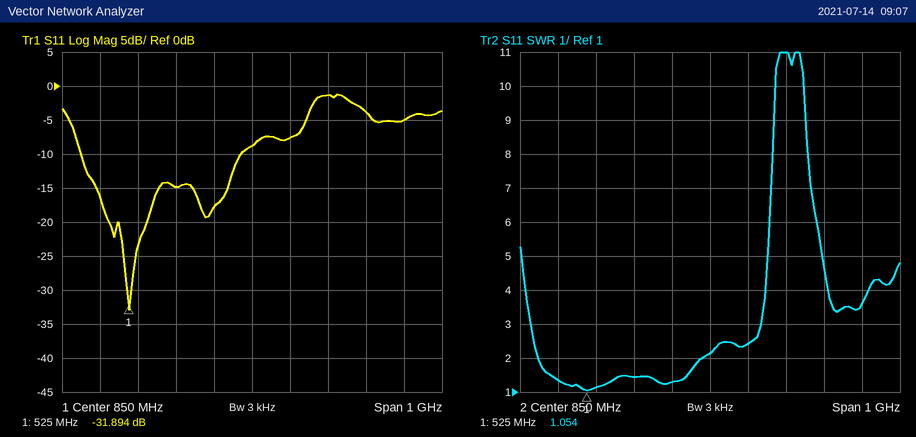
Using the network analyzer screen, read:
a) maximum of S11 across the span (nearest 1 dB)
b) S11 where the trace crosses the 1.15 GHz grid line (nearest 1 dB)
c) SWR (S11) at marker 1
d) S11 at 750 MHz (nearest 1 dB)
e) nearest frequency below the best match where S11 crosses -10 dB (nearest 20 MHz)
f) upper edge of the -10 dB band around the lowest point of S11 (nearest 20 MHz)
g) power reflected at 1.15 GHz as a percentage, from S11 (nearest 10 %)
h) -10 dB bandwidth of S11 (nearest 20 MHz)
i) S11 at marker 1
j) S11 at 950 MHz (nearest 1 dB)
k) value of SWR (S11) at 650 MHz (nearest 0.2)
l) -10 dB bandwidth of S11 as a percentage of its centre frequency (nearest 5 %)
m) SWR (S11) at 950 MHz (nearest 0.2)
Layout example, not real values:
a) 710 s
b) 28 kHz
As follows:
a) -1 dB
b) -4 dB
c) 1.054
d) -18 dB
e) 400 MHz
f) 820 MHz
g) 40 %
h) 420 MHz
i) -31.894 dB
j) -8 dB
k) 1.4
l) 70 %
m) 2.4
